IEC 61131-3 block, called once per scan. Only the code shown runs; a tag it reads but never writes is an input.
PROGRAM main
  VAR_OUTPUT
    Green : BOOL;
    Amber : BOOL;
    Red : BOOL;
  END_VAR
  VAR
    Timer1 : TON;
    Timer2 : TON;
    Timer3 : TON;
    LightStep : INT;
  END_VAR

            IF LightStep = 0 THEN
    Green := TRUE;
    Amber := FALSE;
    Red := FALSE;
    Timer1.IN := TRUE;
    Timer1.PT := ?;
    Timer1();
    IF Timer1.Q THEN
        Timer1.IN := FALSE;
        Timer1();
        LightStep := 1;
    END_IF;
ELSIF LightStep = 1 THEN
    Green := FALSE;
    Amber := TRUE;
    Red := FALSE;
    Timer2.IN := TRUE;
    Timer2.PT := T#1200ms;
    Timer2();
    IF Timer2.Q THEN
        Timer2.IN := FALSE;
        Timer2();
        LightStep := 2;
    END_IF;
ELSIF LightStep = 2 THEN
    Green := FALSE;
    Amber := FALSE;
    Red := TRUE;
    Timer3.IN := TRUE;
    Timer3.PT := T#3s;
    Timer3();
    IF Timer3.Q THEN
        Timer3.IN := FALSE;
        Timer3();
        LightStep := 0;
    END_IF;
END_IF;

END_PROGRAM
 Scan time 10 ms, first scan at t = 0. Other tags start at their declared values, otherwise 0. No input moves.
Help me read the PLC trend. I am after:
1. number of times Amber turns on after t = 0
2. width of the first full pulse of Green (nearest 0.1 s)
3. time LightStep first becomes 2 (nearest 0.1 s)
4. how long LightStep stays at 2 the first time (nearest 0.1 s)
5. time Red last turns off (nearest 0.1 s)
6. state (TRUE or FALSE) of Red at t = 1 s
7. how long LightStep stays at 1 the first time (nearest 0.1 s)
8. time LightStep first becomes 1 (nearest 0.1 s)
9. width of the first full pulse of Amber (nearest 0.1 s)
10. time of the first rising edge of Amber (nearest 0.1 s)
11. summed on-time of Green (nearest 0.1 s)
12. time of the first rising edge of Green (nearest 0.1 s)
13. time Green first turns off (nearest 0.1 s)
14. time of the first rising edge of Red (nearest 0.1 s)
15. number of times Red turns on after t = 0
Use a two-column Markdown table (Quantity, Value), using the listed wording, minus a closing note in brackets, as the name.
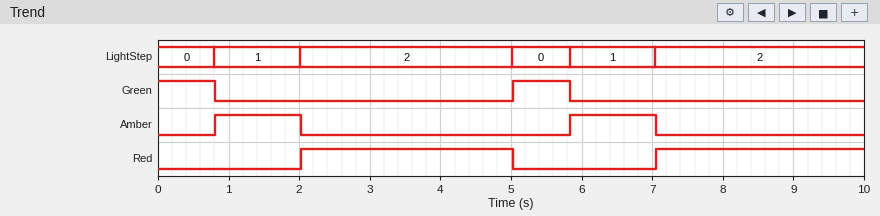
| Quantity | Value |
|---|---|
| number of times Amber turns on after t = 0 | 2 |
| width of the first full pulse of Green | 0.8 s |
| time LightStep first becomes 2 | 2.0 s |
| how long LightStep stays at 2 the first time | 3.0 s |
| time Red last turns off | 5.0 s |
| state (TRUE or FALSE) of Red at t = 1 s | FALSE |
| how long LightStep stays at 1 the first time | 1.2 s |
| time LightStep first becomes 1 | 0.8 s |
| width of the first full pulse of Amber | 1.2 s |
| time of the first rising edge of Amber | 0.8 s |
| summed on-time of Green | 1.6 s |
| time of the first rising edge of Green | 5.0 s |
| time Green first turns off | 0.8 s |
| time of the first rising edge of Red | 2.0 s |
| number of times Red turns on after t = 0 | 2 |
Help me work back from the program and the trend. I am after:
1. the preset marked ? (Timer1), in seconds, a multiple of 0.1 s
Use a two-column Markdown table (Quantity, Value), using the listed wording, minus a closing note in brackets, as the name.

| Quantity | Value |
|---|---|
| the preset marked ? (Timer1), in seconds, a multiple of 0.1 s | 0.8 s |
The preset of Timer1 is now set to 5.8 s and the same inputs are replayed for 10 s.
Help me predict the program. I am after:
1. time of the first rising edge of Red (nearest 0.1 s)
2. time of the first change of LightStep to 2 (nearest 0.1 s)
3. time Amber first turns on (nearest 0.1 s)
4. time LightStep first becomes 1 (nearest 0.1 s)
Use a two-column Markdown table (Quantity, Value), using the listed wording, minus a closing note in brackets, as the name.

| Quantity | Value |
|---|---|
| time of the first rising edge of Red | 7.0 s |
| time of the first change of LightStep to 2 | 7.0 s |
| time Amber first turns on | 5.8 s |
| time LightStep first becomes 1 | 5.8 s |
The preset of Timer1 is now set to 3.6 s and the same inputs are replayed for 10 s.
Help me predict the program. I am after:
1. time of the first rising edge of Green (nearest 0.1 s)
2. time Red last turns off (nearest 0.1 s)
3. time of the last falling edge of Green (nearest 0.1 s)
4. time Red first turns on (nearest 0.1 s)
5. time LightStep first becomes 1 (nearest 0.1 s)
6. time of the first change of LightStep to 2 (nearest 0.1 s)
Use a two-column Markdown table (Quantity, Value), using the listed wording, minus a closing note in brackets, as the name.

| Quantity | Value |
|---|---|
| time of the first rising edge of Green | 7.8 s |
| time Red last turns off | 7.8 s |
| time of the last falling edge of Green | 3.6 s |
| time Red first turns on | 4.8 s |
| time LightStep first becomes 1 | 3.6 s |
| time of the first change of LightStep to 2 | 4.8 s |
